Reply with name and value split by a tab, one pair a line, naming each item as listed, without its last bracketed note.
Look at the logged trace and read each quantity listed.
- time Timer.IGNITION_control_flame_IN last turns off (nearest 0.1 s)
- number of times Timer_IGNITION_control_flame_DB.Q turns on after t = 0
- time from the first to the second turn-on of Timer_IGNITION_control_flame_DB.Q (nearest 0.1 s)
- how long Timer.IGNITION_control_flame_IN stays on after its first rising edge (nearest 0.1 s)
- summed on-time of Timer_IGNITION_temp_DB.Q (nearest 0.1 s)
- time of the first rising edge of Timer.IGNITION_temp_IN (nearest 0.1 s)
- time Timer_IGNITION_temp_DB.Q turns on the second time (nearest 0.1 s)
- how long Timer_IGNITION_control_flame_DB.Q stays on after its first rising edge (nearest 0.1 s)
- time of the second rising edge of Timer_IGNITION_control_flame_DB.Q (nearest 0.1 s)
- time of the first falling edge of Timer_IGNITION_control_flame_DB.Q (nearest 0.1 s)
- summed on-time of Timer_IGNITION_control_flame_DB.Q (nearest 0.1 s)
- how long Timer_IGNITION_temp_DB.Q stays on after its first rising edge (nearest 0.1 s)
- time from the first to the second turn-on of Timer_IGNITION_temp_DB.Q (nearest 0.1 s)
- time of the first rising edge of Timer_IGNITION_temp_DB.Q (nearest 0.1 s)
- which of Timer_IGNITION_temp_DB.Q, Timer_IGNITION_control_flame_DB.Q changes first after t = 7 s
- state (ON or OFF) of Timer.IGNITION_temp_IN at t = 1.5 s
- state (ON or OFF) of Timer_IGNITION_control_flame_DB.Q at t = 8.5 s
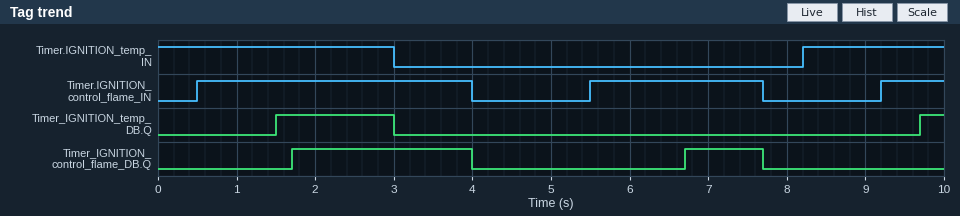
time Timer.IGNITION_control_flame_IN last turns off	7.7 s
number of times Timer_IGNITION_control_flame_DB.Q turns on after t = 0	2
time from the first to the second turn-on of Timer_IGNITION_control_flame_DB.Q	5.0 s
how long Timer.IGNITION_control_flame_IN stays on after its first rising edge	3.5 s
summed on-time of Timer_IGNITION_temp_DB.Q	1.8 s
time of the first rising edge of Timer.IGNITION_temp_IN	8.2 s
time Timer_IGNITION_temp_DB.Q turns on the second time	9.7 s
how long Timer_IGNITION_control_flame_DB.Q stays on after its first rising edge	2.3 s
time of the second rising edge of Timer_IGNITION_control_flame_DB.Q	6.7 s
time of the first falling edge of Timer_IGNITION_control_flame_DB.Q	4.0 s
summed on-time of Timer_IGNITION_control_flame_DB.Q	3.3 s
how long Timer_IGNITION_temp_DB.Q stays on after its first rising edge	1.5 s
time from the first to the second turn-on of Timer_IGNITION_temp_DB.Q	8.2 s
time of the first rising edge of Timer_IGNITION_temp_DB.Q	1.5 s
which of Timer_IGNITION_temp_DB.Q, Timer_IGNITION_control_flame_DB.Q changes first after t = 7 s	Timer_IGNITION_control_flame_DB.Q
state (ON or OFF) of Timer.IGNITION_temp_IN at t = 1.5 s	ON
state (ON or OFF) of Timer_IGNITION_control_flame_DB.Q at t = 8.5 s	OFF
